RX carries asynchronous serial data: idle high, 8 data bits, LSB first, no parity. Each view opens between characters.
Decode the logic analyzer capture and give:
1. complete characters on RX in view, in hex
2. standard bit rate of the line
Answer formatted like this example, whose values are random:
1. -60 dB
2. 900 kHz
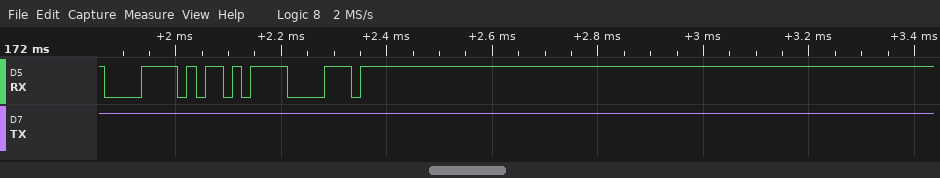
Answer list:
1. 78, EB, B8
2. 57600 baud
